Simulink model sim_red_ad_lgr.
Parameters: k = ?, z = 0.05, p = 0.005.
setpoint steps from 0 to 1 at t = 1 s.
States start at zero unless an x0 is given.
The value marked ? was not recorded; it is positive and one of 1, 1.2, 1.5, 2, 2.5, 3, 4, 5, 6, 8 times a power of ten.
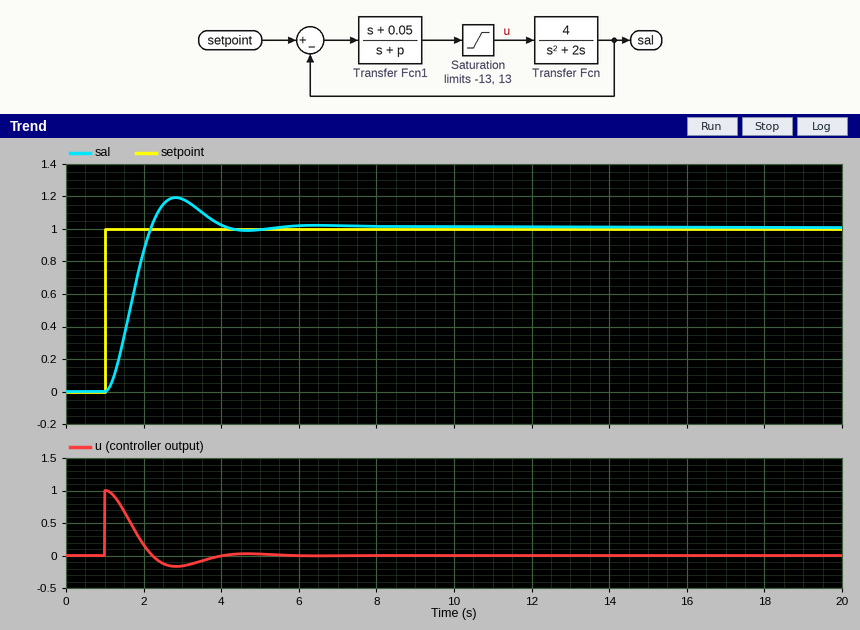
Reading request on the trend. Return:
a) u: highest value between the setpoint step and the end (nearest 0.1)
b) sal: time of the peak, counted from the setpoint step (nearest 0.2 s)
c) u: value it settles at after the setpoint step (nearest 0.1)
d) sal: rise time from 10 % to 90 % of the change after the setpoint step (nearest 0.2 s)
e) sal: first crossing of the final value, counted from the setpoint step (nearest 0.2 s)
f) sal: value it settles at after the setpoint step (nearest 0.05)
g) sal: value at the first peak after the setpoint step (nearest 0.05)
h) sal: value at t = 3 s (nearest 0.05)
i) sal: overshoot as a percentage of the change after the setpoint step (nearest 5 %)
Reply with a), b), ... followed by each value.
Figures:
a) 1.0
b) 1.8 s
c) 0.0
d) 0.8 s
e) 1.2 s
f) 1.00
g) 1.20
h) 1.20
i) 20 %
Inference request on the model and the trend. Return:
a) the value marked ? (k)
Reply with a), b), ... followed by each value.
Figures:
a) 1
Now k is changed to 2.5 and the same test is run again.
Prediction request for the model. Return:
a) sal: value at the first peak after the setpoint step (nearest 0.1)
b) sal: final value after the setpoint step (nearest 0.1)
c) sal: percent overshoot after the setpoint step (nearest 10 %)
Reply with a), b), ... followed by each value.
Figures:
a) 1.4
b) 1.0
c) 40 %
